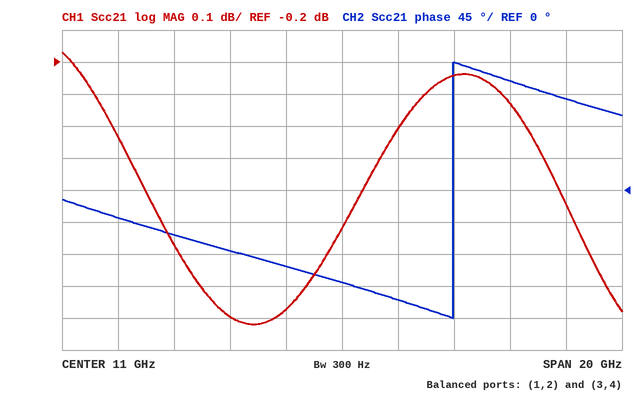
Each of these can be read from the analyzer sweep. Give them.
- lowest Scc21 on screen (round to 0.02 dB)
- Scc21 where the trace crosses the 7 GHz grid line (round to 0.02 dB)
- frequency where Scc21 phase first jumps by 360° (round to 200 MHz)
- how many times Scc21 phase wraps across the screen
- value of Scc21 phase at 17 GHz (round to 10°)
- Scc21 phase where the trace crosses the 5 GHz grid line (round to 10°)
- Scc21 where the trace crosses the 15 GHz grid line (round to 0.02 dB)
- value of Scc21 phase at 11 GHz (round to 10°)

-1.02 dB
-1.00 dB
15.0 GHz
1
150°
-60°
-0.24 dB
-130°
